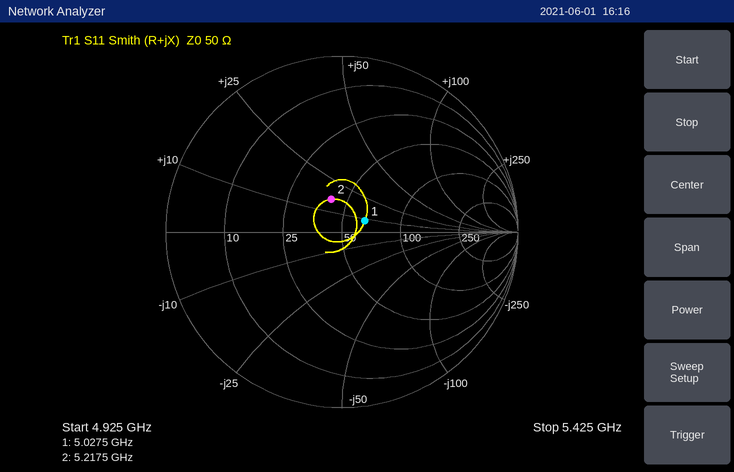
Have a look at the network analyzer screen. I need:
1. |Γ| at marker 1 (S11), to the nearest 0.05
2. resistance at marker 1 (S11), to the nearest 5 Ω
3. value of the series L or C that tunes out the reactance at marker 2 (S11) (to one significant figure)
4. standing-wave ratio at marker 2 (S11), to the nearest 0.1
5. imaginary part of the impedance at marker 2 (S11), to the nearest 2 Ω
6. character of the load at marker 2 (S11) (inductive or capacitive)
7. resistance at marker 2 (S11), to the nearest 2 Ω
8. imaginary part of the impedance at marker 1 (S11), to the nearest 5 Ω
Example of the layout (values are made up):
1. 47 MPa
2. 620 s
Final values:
1. 0.15
2. 65 Ω
3. 2 pF
4. 1.5
5. +16 Ω
6. inductive
7. 42 Ω
8. +10 Ω
